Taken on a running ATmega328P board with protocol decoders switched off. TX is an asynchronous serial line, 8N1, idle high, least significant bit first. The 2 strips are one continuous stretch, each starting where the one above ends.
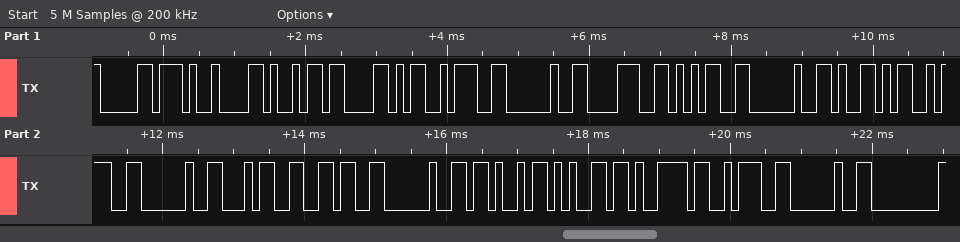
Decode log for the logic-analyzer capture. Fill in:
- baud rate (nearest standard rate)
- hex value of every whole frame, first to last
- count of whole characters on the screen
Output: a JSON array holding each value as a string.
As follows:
["9600 baud", "B0 09 69 58 3A 20 38 35 20 59 3A 20 34 36 20 4B 65 79 3A 20 00", "21"]
